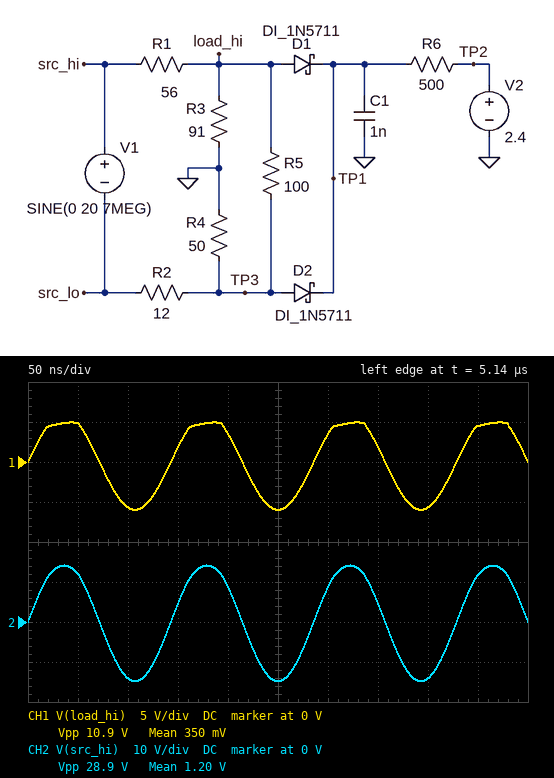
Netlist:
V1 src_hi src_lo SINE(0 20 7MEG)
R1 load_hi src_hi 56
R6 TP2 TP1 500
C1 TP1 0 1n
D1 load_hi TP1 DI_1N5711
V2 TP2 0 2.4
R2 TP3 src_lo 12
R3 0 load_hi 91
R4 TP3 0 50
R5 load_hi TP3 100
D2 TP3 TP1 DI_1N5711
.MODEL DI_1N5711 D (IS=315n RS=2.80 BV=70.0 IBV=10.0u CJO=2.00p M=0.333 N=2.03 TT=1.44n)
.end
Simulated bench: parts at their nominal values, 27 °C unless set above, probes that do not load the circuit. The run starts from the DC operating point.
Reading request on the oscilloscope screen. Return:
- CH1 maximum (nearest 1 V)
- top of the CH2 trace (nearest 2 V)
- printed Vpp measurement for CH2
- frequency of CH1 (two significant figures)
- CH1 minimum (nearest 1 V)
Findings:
5 V
14 V
28.9 V
7.0 MHz
-6 V
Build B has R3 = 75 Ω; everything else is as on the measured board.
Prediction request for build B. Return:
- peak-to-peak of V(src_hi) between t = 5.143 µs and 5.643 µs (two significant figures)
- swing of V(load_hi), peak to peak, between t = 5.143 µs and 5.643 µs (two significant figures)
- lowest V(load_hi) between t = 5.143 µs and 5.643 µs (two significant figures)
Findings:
28 V
10 V
-5.4 V
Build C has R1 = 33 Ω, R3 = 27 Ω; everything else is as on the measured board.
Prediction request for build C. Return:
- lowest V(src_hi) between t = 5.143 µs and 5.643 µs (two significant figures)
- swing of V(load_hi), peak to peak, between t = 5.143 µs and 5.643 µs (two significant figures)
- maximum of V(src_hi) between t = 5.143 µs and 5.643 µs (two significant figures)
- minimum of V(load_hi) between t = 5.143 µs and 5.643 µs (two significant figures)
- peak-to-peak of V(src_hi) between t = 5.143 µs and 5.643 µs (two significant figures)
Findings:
-12 V
7.3 V
11 V
-3.9 V
23 V
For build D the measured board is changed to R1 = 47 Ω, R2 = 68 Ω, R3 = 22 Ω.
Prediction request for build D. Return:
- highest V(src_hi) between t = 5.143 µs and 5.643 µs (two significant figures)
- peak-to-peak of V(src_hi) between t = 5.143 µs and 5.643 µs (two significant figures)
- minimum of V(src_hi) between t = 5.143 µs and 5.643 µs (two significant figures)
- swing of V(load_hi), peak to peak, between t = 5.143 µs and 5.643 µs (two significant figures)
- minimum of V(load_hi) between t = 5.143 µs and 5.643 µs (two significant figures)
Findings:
7.6 V
15 V
-7.8 V
3.3 V
-1.7 V
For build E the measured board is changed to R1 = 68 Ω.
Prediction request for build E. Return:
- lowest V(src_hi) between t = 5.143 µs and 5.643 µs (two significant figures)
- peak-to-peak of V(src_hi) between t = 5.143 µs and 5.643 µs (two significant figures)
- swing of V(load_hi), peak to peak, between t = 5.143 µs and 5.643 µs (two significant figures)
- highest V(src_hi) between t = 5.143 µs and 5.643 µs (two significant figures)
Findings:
-15 V
30 V
10 V
15 V
